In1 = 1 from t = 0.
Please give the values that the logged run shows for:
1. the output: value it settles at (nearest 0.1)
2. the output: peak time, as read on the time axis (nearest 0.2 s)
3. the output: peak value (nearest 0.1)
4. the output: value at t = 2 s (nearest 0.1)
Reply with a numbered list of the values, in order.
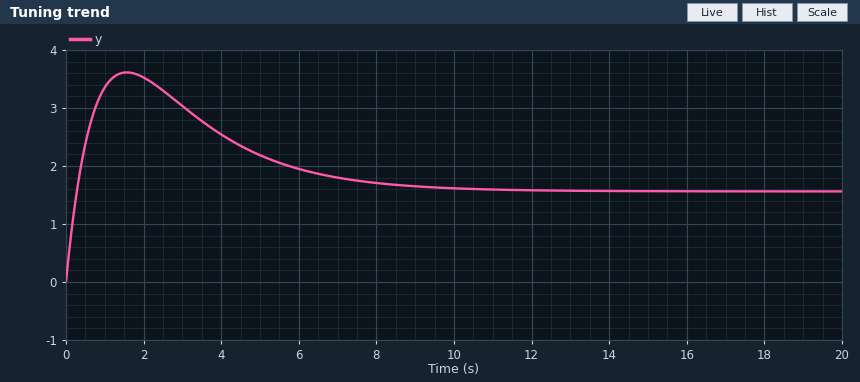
1. 1.6
2. 1.6 s
3. 3.6
4. 3.5
